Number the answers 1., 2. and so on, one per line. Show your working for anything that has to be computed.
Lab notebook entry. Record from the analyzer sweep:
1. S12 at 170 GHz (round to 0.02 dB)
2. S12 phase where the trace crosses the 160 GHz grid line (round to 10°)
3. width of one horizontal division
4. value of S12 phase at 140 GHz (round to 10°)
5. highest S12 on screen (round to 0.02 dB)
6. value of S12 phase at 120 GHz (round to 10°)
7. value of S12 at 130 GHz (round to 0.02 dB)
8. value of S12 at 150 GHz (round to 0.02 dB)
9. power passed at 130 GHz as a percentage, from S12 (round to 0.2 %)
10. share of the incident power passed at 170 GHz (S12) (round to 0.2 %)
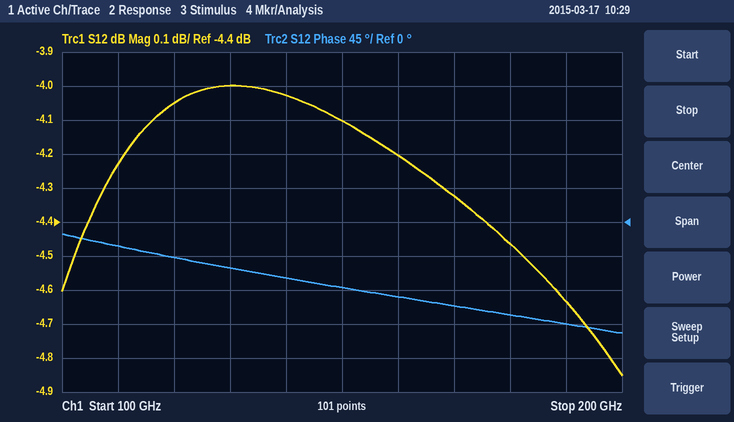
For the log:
1. -4.32 dB
2. -100°
3. 10 GHz
4. -70°
5. -4.00 dB
6. -50°
7. -4.00 dB
8. -4.10 dB
9. 10^(-4/10) ≈ 39.8 %
10. 10^(-4.32/10) ≈ 37.0 %
